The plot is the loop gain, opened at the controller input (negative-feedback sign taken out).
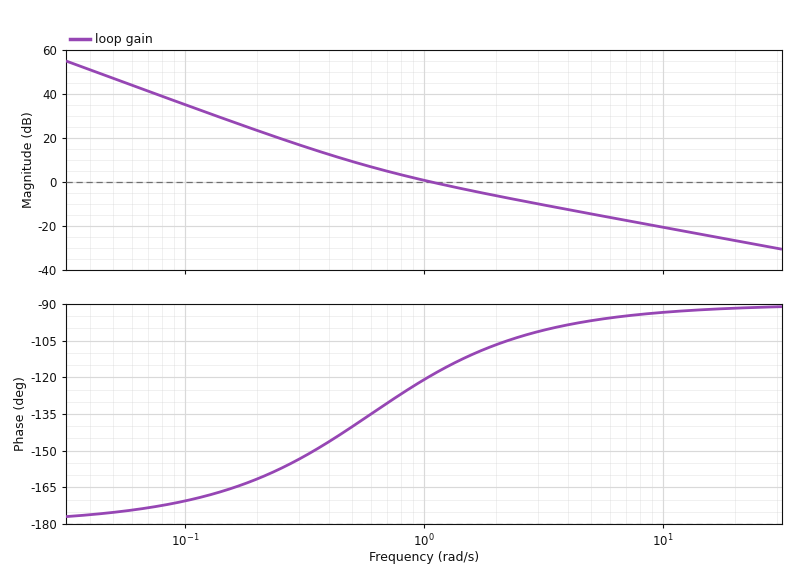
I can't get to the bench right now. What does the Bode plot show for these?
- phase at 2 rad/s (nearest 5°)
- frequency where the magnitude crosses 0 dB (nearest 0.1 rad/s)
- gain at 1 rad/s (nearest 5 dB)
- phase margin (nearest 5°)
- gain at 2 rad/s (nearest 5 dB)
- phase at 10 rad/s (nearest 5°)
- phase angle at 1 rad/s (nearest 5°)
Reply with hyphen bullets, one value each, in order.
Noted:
- -105°
- 1.1 rad/s
- 0 dB
- 60°
- -5 dB
- -95°
- -120°
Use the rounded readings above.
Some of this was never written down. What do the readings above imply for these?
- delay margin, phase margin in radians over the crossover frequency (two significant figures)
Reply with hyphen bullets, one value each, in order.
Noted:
- 0.95 s
